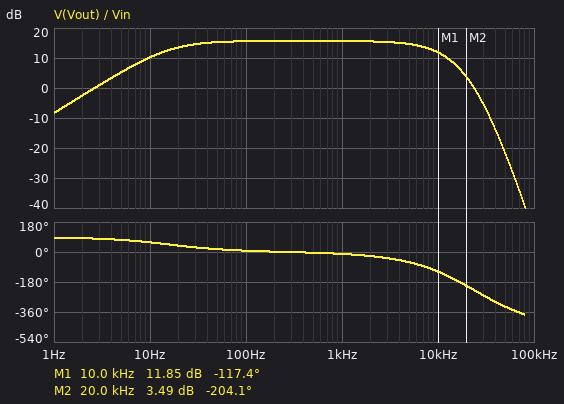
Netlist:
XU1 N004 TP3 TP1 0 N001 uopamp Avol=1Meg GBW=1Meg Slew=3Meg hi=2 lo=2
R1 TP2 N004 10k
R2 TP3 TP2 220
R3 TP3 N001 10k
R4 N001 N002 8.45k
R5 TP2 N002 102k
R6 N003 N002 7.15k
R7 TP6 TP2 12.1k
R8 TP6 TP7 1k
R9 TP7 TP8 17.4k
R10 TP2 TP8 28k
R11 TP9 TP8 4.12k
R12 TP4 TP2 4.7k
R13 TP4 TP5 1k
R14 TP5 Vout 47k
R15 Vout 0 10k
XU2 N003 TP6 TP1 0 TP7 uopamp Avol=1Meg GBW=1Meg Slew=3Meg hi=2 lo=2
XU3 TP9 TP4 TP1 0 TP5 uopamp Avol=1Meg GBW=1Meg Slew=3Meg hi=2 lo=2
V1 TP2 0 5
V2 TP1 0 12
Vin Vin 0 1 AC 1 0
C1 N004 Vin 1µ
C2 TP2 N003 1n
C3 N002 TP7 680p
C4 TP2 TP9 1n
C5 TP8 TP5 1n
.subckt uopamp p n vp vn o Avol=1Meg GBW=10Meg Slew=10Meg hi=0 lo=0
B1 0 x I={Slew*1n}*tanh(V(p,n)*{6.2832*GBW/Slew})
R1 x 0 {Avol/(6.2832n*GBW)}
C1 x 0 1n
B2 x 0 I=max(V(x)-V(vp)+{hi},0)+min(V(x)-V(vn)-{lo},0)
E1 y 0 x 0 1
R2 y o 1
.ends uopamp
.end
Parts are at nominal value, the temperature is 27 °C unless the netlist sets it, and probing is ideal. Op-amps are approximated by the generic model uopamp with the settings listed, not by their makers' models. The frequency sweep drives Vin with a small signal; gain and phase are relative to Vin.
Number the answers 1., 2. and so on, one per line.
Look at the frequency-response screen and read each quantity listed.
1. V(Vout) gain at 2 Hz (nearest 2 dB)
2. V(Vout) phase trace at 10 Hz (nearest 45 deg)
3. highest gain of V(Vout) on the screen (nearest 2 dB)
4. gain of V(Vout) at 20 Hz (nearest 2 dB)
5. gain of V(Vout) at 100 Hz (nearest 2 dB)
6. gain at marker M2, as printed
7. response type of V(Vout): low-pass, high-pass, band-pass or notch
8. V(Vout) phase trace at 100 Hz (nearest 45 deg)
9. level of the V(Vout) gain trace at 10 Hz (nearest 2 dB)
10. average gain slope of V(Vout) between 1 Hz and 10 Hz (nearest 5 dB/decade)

1. -2 dB
2. 45 deg
3. 16 dB
4. 14 dB
5. 16 dB
6. 3.49 dB
7. band-pass
8. 0 deg
9. 10 dB
10. 20 dB/decade
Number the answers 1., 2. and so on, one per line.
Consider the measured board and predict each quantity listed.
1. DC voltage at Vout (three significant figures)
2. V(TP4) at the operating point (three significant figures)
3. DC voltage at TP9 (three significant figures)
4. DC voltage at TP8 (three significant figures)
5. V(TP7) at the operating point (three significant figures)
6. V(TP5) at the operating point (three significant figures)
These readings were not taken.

1. 877 mV
2. 5.00 V
3. 5.00 V
4. 5.00 V
5. 5.00 V
6. 5.00 V
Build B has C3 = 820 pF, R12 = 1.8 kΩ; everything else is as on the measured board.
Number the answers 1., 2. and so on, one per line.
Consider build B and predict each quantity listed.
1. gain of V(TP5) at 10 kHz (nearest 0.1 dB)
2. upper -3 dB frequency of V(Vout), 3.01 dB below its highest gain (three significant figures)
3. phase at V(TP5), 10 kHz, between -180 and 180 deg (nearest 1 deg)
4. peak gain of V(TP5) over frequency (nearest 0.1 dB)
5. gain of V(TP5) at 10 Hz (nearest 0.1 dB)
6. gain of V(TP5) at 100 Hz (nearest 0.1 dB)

1. 30.6 dB
2. 11.2 kHz
3. -109 deg
4. 33.0 dB
5. 27.5 dB
6. 32.9 dB
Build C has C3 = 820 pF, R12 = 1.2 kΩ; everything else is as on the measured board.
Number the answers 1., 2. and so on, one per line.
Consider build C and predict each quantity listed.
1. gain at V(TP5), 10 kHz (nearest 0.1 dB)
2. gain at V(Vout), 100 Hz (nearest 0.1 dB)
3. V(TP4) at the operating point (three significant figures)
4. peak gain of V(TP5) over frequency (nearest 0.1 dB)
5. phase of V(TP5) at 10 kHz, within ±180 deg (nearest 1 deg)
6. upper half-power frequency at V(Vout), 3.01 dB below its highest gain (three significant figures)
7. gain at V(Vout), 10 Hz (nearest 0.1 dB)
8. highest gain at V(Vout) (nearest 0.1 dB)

1. 32.9 dB
2. 19.2 dB
3. 5.00 V
4. 34.4 dB
5. -99 deg
6. 14.9 kHz
7. 13.8 dB
8. 19.3 dB
